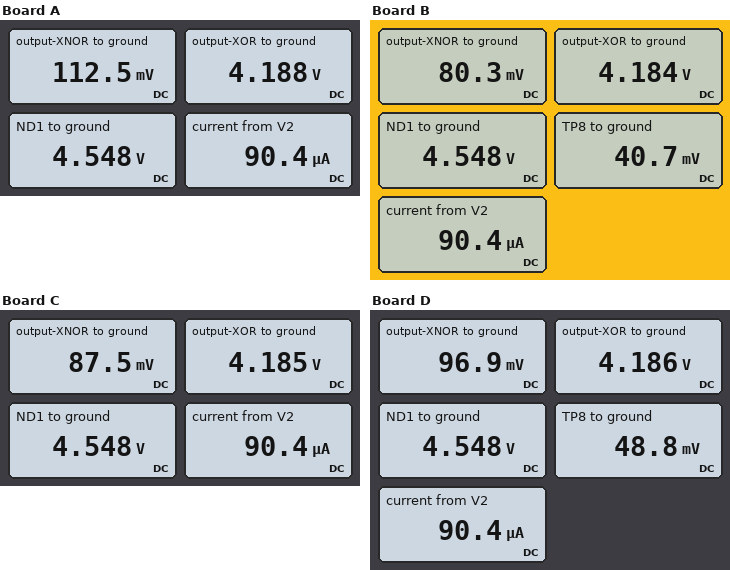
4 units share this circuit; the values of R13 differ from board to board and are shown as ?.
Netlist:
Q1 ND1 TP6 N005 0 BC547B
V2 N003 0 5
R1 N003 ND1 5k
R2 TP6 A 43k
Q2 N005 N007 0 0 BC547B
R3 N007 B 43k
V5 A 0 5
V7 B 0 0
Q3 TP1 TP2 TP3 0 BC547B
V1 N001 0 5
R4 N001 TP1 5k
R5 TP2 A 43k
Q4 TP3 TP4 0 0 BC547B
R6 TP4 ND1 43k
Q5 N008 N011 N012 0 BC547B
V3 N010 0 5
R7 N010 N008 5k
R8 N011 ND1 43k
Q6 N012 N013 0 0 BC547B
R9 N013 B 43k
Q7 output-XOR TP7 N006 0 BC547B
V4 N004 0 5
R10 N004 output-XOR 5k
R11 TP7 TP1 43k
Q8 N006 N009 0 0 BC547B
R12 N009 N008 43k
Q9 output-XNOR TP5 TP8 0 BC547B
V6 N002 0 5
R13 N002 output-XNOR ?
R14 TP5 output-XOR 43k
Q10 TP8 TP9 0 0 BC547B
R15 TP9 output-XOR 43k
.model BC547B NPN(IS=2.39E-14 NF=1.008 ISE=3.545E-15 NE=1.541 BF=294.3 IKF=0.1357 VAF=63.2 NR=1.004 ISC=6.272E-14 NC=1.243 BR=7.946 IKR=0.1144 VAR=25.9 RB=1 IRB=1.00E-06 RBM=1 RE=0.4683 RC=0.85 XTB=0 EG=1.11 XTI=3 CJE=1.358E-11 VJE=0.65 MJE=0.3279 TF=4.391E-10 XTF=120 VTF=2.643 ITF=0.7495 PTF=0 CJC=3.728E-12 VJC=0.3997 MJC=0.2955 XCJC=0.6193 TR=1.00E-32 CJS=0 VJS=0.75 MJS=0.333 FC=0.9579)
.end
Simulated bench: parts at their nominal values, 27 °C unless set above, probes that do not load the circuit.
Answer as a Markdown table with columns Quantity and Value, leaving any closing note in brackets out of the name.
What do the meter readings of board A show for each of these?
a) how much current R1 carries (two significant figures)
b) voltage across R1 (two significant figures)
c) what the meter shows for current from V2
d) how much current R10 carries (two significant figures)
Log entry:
| Quantity | Value |
|---|---|
| how much current R1 carries | 90 µA |
| voltage across R1 | 450 mV |
| what the meter shows for current from V2 | 90.4 µA |
| how much current R10 carries | 160 µA |
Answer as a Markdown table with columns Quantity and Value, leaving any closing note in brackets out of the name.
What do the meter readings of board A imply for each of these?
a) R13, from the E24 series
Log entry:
| Quantity | Value |
|---|---|
| R13, from the E24 series | 2 kΩ |
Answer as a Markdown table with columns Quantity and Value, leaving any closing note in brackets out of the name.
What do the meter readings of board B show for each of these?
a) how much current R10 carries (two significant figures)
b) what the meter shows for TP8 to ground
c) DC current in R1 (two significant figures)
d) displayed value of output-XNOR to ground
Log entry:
| Quantity | Value |
|---|---|
| how much current R10 carries | 160 µA |
| what the meter shows for TP8 to ground | 40.7 mV |
| DC current in R1 | 90 µA |
| displayed value of output-XNOR to ground | 80.3 mV |
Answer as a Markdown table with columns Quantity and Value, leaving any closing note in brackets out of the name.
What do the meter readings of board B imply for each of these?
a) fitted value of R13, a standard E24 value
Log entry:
| Quantity | Value |
|---|---|
| fitted value of R13, a standard E24 value | 3.9 kΩ |
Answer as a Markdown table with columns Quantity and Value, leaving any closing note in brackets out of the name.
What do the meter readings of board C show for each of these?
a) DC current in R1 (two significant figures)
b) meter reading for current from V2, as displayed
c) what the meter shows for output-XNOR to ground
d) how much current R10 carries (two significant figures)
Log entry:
| Quantity | Value |
|---|---|
| DC current in R1 | 90 µA |
| meter reading for current from V2, as displayed | 90.4 µA |
| what the meter shows for output-XNOR to ground | 87.5 mV |
| how much current R10 carries | 160 µA |
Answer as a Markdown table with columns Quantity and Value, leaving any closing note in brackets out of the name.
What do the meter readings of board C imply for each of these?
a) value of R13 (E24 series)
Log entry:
| Quantity | Value |
|---|---|
| value of R13 | 3.3 kΩ |
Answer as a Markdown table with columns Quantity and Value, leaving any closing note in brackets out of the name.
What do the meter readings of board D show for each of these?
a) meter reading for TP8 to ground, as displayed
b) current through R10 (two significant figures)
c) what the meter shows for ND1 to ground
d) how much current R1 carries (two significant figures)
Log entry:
| Quantity | Value |
|---|---|
| meter reading for TP8 to ground, as displayed | 48.8 mV |
| current through R10 | 160 µA |
| what the meter shows for ND1 to ground | 4.548 V |
| how much current R1 carries | 90 µA |
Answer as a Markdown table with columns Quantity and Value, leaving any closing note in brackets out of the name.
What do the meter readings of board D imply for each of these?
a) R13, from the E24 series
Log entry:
| Quantity | Value |
|---|---|
| R13, from the E24 series | 2.7 kΩ |
